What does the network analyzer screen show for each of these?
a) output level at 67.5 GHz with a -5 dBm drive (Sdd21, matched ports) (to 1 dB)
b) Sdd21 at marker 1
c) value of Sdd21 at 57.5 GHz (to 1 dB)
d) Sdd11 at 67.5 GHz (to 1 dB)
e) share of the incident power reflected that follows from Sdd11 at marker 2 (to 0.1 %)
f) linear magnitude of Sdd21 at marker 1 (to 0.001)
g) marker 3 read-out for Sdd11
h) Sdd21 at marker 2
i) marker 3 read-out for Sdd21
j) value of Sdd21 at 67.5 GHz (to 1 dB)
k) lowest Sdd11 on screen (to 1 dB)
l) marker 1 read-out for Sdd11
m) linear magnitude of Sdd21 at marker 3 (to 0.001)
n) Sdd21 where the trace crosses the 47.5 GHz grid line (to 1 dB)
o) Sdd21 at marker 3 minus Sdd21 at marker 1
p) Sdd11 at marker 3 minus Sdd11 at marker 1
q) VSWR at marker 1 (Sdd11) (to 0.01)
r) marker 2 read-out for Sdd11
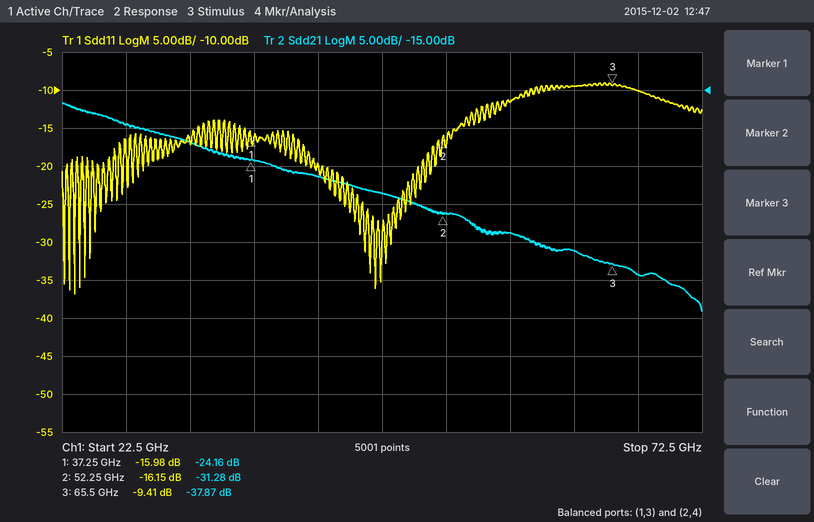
-44 dBm
-24.16 dB
-34 dB
-10 dB
2.4 %
0.062
-9.41 dB
-31.28 dB
-37.87 dB
-39 dB
-37 dB
-15.98 dB
0.013
-29 dB
-13.71 dB
6.57 dB
1.38
-16.15 dB
